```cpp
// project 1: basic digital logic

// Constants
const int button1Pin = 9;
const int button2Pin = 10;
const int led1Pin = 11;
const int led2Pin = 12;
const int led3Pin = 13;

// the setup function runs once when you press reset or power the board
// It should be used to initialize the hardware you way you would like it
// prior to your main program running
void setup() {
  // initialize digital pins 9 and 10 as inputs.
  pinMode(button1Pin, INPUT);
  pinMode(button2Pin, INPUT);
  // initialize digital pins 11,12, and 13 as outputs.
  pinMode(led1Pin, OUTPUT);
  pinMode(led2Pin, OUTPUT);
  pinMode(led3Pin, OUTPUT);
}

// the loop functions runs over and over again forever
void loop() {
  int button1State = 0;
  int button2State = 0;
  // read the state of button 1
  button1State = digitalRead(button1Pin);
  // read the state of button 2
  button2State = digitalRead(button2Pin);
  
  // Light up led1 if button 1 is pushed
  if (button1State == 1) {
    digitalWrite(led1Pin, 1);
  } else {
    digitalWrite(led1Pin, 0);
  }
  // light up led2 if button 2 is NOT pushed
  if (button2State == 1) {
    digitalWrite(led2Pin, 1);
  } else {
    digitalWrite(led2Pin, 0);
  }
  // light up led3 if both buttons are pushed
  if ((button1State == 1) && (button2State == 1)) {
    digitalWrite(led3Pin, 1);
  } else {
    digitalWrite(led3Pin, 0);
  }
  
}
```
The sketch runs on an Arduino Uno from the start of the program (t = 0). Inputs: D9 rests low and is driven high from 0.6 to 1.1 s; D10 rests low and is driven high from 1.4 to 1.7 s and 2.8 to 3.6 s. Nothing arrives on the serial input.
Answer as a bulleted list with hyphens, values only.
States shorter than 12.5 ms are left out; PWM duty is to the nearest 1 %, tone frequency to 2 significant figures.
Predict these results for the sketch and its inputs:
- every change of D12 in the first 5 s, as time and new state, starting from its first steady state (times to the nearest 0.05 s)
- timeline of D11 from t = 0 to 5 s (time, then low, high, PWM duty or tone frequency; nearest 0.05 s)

- 0 s low; 1.4 s high; 1.7 s low; 2.8 s high; 3.6 s low
- 0 s low; 0.6 s high; 1.1 s low
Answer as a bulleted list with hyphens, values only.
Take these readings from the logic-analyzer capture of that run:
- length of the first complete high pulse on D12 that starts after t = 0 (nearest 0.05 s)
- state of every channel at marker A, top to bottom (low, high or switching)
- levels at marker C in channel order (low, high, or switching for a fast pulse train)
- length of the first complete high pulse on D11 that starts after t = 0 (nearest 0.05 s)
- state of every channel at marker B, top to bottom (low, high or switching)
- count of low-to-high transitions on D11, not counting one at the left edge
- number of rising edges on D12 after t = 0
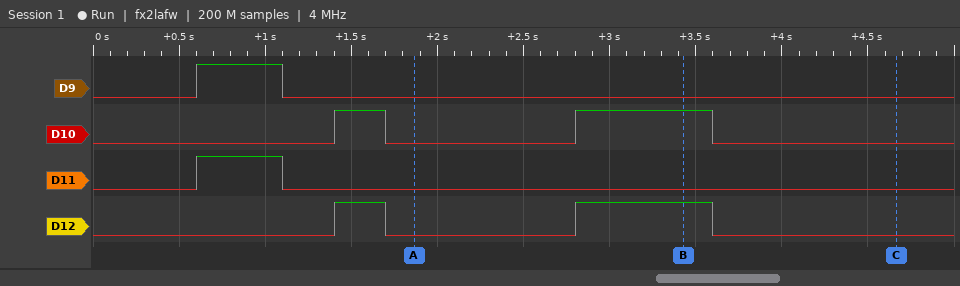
- 0.30 s
- D9 low, D10 low, D11 low, D12 low
- D9 low, D10 low, D11 low, D12 low
- 0.50 s
- D9 low, D10 high, D11 low, D12 high
- 1
- 2
